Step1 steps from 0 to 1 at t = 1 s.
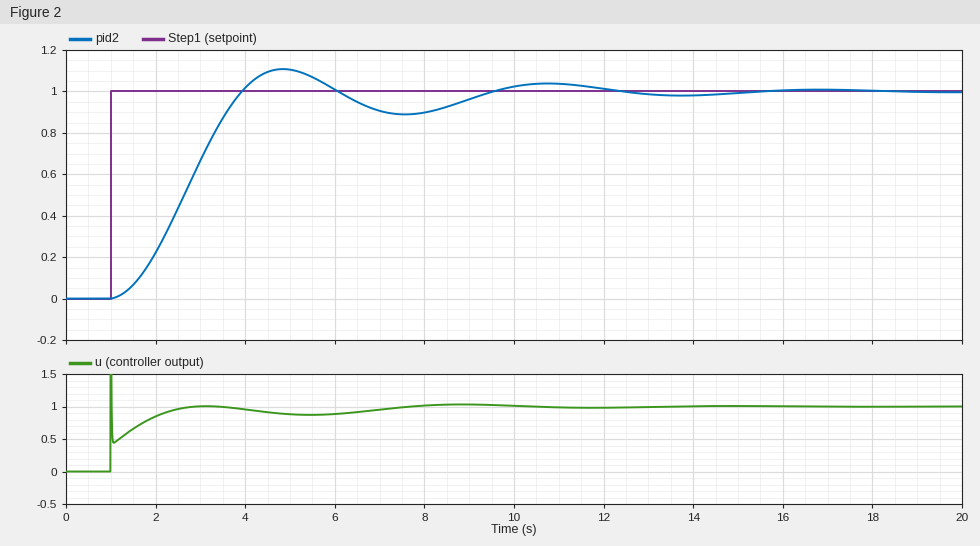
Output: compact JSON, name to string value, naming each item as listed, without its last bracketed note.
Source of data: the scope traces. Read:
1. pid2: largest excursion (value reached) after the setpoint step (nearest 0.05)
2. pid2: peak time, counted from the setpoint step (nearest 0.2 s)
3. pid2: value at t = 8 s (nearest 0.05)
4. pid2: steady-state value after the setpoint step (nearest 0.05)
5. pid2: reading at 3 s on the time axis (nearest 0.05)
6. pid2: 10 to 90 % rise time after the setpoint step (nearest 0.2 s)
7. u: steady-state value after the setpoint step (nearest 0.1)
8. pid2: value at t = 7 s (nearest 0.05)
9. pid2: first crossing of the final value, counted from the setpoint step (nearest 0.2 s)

{"pid2: largest excursion (value reached) after the setpoint step": "1.10", "pid2: peak time, counted from the setpoint step": "3.8 s", "pid2: value at t = 8 s": "0.90", "pid2: steady-state value after the setpoint step": "1.00", "pid2: reading at 3 s on the time axis": "0.65", "pid2: 10 to 90 % rise time after the setpoint step": "2.0 s", "u: steady-state value after the setpoint step": "1.0", "pid2: value at t = 7 s": "0.90", "pid2: first crossing of the final value, counted from the setpoint step": "3.0 s"}
